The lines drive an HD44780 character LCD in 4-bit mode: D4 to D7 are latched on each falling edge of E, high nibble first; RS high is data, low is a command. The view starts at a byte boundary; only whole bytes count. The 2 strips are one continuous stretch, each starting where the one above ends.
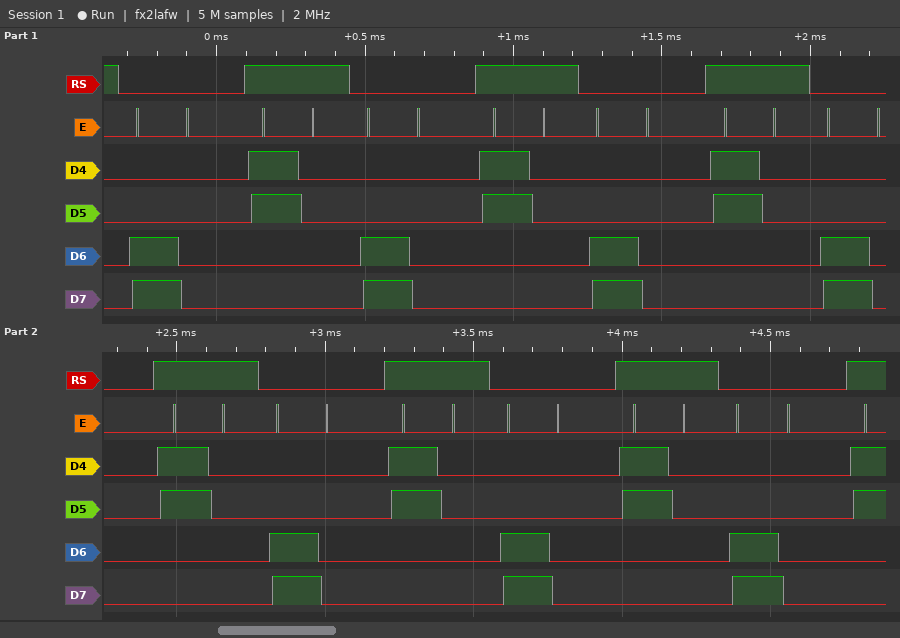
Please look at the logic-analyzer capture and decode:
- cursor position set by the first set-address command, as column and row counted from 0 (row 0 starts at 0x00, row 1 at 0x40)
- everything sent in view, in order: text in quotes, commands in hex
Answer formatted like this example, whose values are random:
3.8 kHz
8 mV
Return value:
column 0, row 1
0xC0 "0" 0xC0 "0" 0xC0 "0" 0xC0 "0" 0xC0 "0" 0xC0 "0" 0xC0
